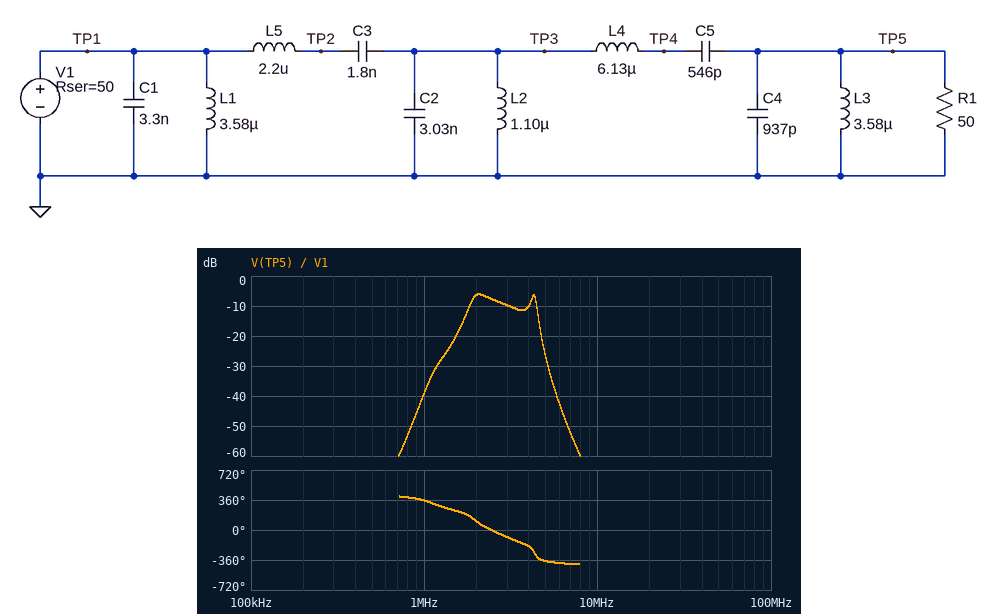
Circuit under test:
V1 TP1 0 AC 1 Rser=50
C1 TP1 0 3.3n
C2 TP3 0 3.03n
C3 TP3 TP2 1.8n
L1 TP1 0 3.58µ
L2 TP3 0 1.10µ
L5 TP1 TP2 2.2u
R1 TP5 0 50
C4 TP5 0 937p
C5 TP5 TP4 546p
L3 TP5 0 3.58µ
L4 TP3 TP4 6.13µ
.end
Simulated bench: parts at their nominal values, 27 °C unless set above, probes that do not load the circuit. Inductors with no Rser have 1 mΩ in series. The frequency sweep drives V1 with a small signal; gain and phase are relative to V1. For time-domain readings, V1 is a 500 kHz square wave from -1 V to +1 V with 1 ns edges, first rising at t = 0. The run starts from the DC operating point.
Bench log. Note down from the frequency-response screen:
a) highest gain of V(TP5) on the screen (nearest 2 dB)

-6 dB
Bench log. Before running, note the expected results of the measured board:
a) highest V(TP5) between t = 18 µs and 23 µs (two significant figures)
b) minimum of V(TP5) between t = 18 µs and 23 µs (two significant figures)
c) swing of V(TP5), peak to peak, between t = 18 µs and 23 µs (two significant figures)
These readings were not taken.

200 mV
-200 mV
400 mV
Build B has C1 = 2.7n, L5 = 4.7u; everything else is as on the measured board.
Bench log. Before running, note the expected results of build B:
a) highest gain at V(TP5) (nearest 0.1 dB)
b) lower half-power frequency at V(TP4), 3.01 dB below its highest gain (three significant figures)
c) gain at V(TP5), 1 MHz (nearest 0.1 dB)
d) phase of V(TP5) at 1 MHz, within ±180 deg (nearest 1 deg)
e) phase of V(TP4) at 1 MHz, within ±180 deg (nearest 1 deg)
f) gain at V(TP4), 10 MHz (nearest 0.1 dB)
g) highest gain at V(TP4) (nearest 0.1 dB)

-7.1 dB
1.76 MHz
-36.5 dB
-9 deg
-159 deg
-69.4 dB
1.7 dB
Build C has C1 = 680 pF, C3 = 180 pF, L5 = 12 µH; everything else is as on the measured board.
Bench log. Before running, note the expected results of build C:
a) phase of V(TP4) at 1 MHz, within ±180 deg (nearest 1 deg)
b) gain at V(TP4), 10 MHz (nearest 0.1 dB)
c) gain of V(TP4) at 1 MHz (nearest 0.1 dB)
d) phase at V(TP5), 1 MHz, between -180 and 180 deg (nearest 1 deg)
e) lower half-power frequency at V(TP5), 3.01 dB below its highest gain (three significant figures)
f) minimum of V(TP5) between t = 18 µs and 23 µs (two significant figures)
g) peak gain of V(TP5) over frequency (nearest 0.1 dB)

-118 deg
-65.0 dB
-45.2 dB
33 deg
2.70 MHz
-170 mV
-6.6 dB
